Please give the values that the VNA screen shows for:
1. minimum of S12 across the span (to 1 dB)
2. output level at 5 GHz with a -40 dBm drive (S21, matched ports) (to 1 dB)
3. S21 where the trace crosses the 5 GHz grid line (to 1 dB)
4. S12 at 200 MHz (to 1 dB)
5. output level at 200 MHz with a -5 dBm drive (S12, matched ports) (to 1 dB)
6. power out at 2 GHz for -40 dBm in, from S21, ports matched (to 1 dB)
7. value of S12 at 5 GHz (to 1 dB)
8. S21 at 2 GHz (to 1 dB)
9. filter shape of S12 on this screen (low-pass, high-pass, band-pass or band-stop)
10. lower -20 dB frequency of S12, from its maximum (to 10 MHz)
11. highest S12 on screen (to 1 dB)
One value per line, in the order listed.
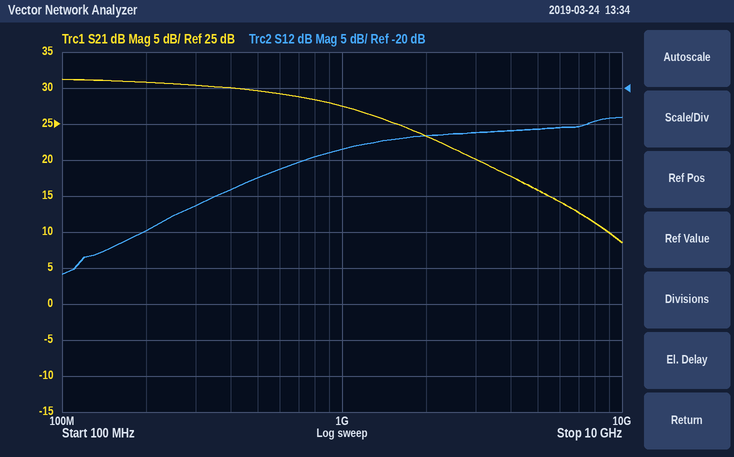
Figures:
-46 dB
-24 dBm
16 dB
-40 dB
-45 dBm
-17 dBm
-26 dB
23 dB
high-pass
120 MHz
-24 dB
